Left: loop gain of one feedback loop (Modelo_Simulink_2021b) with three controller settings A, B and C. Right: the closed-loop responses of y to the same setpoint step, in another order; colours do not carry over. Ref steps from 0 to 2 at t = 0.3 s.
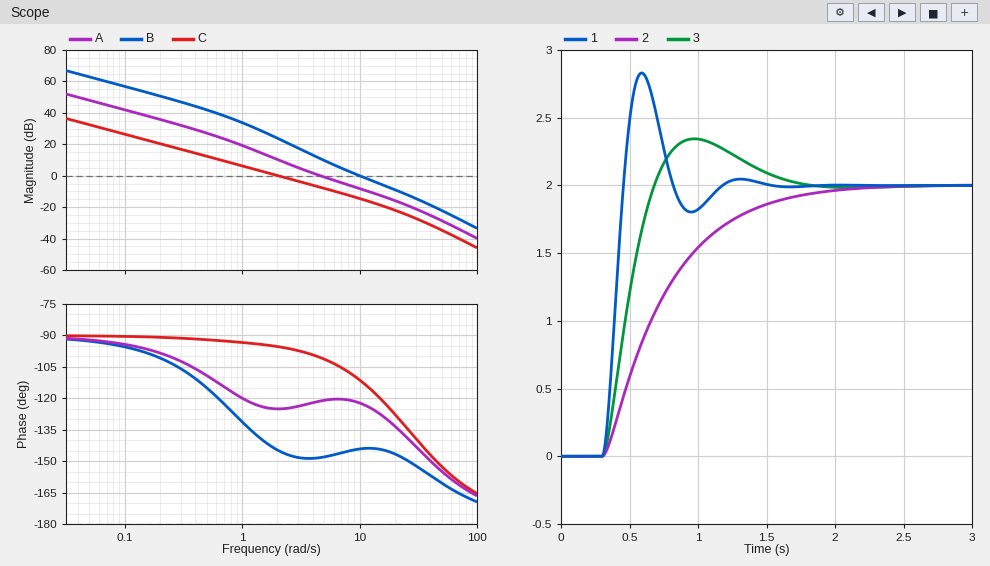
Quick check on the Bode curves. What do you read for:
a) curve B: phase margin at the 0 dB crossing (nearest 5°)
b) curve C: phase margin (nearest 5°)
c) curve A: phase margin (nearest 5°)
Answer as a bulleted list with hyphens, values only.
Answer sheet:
- 35°
- 85°
- 60°
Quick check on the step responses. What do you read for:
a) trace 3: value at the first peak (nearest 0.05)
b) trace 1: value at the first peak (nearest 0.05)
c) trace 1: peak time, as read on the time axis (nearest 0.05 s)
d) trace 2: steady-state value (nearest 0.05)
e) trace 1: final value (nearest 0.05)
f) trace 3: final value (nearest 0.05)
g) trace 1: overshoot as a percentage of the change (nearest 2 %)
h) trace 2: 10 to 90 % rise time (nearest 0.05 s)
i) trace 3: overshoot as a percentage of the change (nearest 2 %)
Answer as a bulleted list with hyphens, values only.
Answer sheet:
- 2.35
- 2.85
- 0.60 s
- 2.00
- 2.00
- 2.00
- 42 %
- 0.95 s
- 18 %
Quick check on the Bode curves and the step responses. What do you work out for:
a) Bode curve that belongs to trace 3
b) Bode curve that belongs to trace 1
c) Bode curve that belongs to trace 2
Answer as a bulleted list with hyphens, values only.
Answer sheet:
- A
- B
- C
